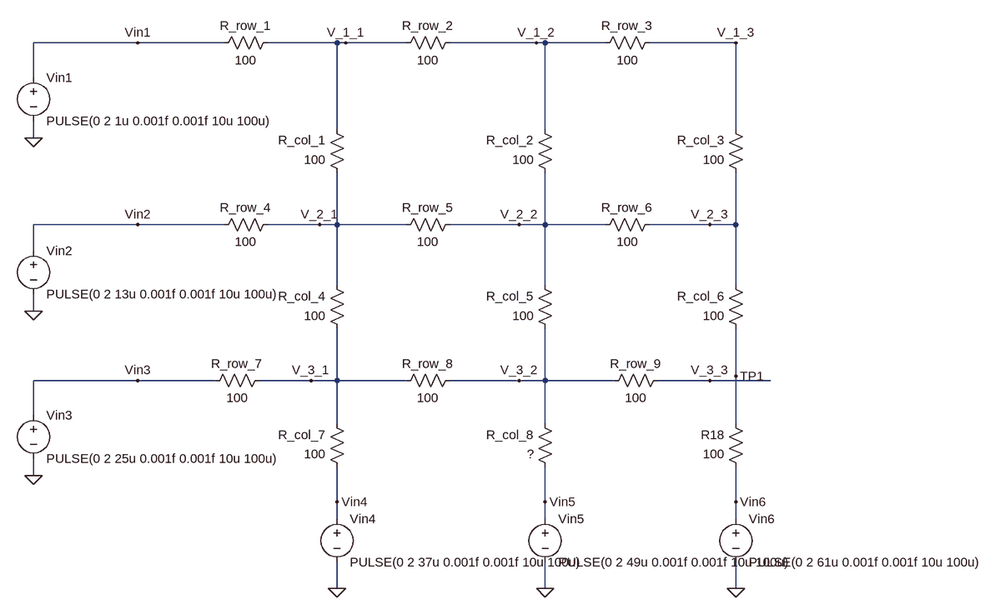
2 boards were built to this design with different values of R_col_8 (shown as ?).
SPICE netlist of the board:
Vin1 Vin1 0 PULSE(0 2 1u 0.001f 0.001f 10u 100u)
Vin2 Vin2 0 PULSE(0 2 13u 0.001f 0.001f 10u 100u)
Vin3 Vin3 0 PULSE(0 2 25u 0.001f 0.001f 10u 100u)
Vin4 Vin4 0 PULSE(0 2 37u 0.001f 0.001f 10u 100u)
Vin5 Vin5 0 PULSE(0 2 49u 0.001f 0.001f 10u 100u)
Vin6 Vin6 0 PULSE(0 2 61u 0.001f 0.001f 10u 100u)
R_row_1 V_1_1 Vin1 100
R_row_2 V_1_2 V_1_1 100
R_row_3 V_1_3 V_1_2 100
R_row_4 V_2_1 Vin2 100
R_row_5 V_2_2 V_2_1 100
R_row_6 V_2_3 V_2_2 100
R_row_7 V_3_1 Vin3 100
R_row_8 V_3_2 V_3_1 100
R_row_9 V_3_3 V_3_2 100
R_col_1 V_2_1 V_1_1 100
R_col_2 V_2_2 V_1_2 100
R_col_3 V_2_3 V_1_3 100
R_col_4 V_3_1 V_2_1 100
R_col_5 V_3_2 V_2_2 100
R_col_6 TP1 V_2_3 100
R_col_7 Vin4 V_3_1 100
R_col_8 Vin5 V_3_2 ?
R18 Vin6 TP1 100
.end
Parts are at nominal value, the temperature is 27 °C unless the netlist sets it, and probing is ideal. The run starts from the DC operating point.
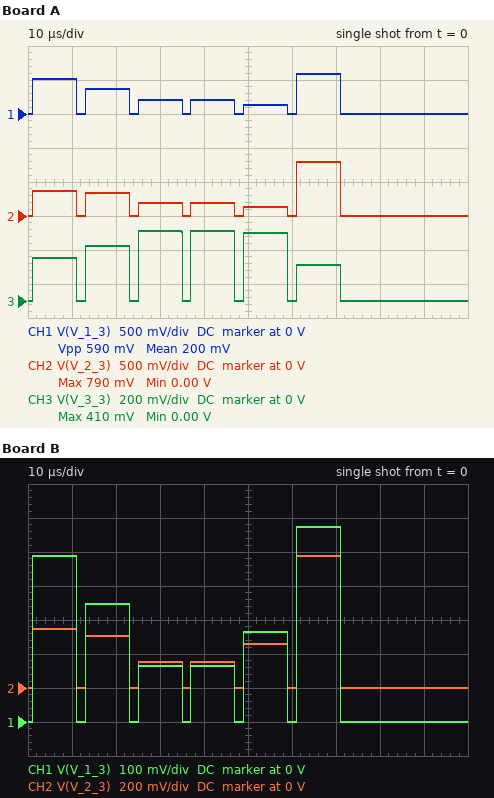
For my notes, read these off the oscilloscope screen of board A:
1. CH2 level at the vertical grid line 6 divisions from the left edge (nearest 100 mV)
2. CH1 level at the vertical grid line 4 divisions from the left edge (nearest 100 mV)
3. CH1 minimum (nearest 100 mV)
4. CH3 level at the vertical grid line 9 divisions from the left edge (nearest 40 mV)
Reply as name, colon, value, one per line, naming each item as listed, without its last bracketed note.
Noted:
CH2 level at the vertical grid line 6 divisions from the left edge: 0 V
CH1 level at the vertical grid line 4 divisions from the left edge: 200 mV
CH1 minimum: 0 V
CH3 level at the vertical grid line 9 divisions from the left edge: 0 V
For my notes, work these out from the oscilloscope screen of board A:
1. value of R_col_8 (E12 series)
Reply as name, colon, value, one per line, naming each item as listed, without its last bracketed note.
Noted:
value of R_col_8: 330 Ω
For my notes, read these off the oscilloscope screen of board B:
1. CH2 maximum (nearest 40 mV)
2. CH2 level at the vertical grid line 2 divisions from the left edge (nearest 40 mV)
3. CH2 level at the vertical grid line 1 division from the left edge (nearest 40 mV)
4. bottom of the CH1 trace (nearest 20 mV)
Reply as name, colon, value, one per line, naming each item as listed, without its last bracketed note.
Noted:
CH2 maximum: 760 mV
CH2 level at the vertical grid line 2 divisions from the left edge: 320 mV
CH2 level at the vertical grid line 1 division from the left edge: 360 mV
bottom of the CH1 trace: 0 V
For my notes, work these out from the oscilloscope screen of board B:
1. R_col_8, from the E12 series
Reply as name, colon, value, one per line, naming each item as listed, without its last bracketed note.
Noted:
R_col_8, from the E12 series: 120 Ω
